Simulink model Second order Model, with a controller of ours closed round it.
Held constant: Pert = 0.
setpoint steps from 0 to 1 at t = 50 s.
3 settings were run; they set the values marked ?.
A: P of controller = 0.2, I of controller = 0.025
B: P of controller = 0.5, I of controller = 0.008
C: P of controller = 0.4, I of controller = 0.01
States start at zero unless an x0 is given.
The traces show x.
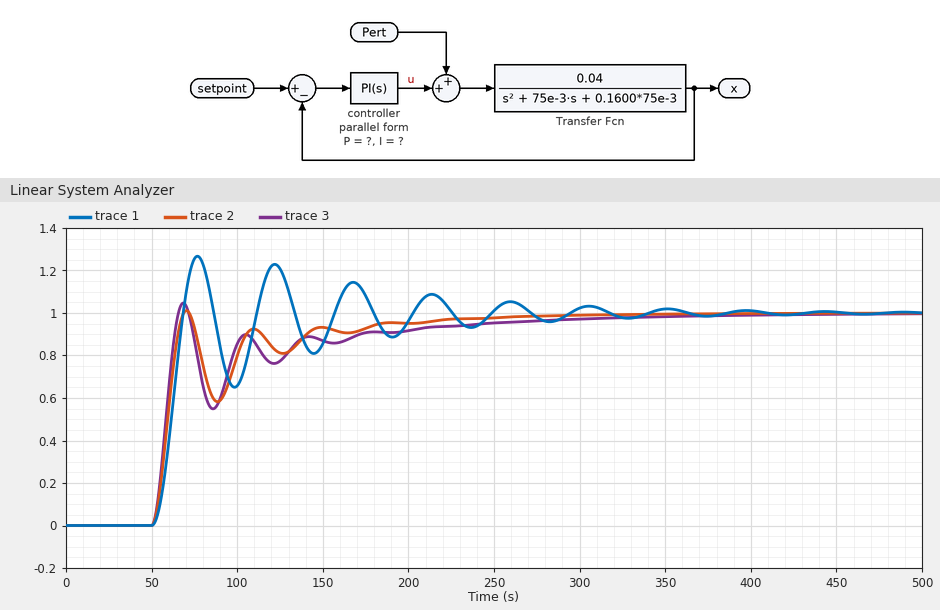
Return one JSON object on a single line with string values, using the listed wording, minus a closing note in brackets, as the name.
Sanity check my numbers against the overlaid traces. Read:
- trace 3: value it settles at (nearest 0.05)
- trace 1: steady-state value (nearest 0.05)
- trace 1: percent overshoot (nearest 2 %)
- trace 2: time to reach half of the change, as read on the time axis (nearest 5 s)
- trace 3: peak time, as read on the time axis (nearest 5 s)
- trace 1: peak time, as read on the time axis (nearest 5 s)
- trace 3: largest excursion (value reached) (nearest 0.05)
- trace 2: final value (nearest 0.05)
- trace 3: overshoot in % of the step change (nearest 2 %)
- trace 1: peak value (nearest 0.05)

{"trace 3: value it settles at": "1.00", "trace 1: steady-state value": "1.00", "trace 1: percent overshoot": "26 %", "trace 2: time to reach half of the change, as read on the time axis": "60 s", "trace 3: peak time, as read on the time axis": "70 s", "trace 1: peak time, as read on the time axis": "75 s", "trace 3: largest excursion (value reached)": "1.05", "trace 2: final value": "1.00", "trace 3: overshoot in % of the step change": "4 %", "trace 1: peak value": "1.25"}
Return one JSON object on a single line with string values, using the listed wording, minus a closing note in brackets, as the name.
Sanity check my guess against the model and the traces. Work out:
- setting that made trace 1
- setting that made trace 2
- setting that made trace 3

{"setting that made trace 1": "A", "setting that made trace 2": "C", "setting that made trace 3": "B"}
